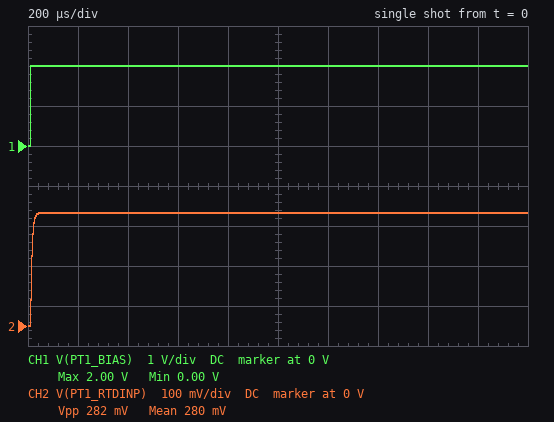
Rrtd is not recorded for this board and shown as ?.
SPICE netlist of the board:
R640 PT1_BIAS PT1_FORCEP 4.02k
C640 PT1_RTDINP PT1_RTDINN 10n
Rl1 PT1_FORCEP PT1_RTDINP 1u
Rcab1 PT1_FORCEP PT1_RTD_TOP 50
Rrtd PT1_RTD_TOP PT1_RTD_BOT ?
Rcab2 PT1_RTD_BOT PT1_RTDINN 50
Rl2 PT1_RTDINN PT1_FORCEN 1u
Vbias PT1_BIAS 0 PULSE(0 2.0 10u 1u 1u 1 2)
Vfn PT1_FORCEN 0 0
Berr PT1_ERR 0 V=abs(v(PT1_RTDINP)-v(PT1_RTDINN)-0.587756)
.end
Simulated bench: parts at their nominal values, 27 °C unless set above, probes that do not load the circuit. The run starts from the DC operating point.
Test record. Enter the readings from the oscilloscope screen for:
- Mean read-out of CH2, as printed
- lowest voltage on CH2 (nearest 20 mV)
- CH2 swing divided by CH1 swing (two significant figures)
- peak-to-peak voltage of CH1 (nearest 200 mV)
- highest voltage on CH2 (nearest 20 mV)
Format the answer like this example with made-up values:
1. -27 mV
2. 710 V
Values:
1. 280 mV
2. 0 V
3. 0.14
4. 2.0 V
5. 280 mV
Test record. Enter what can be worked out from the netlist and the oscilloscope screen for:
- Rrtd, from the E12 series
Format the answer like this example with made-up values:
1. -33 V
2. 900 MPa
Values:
1. 560 Ω
